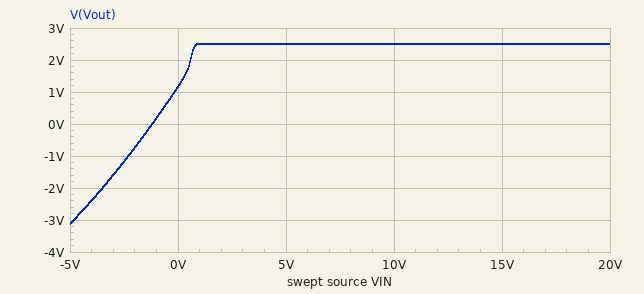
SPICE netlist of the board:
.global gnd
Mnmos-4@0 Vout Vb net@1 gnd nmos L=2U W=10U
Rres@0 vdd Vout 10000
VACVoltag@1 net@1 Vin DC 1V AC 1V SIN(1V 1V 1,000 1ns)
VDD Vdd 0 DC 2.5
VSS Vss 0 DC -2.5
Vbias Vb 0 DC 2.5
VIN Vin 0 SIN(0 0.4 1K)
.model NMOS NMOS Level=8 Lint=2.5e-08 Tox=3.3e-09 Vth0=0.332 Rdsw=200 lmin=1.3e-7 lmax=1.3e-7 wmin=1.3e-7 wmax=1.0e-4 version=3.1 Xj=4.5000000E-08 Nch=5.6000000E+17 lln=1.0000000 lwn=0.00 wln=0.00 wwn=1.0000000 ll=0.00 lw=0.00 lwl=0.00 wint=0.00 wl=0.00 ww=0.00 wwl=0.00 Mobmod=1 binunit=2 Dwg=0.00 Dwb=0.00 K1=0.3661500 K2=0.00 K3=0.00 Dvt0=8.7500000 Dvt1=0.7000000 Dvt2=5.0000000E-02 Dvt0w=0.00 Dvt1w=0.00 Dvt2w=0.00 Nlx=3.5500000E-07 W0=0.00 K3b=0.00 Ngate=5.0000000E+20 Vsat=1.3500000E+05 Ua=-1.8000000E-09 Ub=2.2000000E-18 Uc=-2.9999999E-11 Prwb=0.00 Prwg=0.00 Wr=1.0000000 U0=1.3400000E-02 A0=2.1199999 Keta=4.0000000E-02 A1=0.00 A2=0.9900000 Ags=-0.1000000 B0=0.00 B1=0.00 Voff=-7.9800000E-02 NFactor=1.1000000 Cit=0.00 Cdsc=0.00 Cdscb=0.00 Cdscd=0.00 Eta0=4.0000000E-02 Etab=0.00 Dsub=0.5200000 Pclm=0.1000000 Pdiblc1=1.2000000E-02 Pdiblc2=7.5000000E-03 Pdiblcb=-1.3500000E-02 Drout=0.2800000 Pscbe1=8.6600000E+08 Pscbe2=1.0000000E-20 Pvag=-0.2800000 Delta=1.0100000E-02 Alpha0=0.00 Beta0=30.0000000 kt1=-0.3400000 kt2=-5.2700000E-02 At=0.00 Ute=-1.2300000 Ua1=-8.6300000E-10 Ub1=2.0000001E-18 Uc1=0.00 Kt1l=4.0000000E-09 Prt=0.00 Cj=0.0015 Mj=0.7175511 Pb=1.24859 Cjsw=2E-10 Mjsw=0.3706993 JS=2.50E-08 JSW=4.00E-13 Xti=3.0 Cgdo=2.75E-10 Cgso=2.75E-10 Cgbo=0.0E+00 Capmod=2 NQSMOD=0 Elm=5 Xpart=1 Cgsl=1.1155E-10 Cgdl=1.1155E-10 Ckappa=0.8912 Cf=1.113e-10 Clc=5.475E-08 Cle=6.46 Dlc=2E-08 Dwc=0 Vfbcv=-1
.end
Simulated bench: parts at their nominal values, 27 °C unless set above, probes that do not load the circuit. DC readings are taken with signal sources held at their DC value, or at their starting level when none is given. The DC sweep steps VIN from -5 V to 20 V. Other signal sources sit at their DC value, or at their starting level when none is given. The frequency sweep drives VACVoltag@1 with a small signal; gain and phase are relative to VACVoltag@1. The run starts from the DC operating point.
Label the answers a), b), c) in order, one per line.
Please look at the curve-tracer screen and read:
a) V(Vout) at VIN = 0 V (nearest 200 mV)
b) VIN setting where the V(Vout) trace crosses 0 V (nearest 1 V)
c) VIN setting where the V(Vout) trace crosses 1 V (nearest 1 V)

a) 1.2 V
b) -1 V
c) 0 V
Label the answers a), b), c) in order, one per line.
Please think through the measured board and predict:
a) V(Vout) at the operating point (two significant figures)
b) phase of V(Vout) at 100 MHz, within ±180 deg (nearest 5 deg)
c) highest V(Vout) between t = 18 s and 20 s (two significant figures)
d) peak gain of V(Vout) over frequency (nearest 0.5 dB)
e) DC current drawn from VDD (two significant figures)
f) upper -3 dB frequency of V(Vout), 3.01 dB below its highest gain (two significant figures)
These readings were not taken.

a) 1.2 V
b) -5 deg
c) 2.5 V
d) 0.5 dB
e) 130 µA
f) 800 MHz
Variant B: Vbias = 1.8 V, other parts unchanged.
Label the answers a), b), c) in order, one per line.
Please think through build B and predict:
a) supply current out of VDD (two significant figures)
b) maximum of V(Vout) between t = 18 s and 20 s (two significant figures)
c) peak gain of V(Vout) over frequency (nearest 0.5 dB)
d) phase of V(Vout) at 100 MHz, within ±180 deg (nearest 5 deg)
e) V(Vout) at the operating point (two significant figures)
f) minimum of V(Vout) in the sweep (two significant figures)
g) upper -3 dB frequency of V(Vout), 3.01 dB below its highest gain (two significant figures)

a) 38 µA
b) 2.5 V
c) 9.0 dB
d) 0 deg
e) 2.1 V
f) -3.2 V
g) 2.7 GHz
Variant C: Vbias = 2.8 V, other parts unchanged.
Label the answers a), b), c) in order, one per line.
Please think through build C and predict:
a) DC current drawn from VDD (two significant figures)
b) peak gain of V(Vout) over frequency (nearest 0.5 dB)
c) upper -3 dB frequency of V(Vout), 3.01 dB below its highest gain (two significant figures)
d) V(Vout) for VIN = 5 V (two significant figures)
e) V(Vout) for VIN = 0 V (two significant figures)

a) 140 µA
b) 0 dB
c) 990 MHz
d) 2.5 V
e) 1.1 V
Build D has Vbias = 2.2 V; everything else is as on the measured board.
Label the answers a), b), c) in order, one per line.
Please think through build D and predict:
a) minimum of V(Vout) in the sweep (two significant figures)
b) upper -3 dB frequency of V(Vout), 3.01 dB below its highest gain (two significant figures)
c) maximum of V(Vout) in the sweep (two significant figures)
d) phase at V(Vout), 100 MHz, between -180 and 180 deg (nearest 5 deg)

a) -3.2 V
b) 540 MHz
c) 2.5 V
d) -10 deg
